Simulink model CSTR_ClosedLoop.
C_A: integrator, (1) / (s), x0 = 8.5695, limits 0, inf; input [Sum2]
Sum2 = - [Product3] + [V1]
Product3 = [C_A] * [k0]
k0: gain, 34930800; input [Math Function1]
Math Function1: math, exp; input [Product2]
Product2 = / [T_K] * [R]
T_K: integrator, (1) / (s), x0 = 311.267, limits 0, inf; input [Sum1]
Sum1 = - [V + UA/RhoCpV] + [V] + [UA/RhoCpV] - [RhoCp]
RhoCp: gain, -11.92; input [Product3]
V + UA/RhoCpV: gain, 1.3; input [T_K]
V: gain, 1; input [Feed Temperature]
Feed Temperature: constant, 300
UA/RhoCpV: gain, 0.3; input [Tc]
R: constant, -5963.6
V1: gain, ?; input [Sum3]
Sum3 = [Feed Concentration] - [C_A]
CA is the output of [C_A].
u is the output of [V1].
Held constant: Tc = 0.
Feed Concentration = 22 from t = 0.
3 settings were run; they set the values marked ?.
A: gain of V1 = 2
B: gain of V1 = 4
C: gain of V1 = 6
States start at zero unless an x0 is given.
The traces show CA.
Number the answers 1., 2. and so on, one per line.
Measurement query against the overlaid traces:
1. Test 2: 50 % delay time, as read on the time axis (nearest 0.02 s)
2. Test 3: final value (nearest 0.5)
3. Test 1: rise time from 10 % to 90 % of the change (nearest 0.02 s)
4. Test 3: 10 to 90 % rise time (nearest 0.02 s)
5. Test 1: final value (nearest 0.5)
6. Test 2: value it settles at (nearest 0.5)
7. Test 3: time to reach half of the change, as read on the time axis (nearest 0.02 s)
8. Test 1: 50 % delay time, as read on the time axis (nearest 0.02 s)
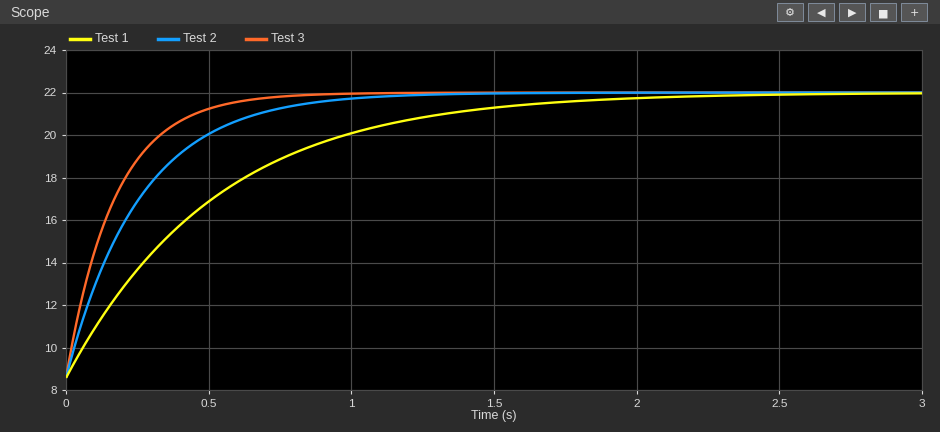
1. 0.18 s
2. 22.0
3. 1.12 s
4. 0.38 s
5. 22.0
6. 22.0
7. 0.12 s
8. 0.36 s
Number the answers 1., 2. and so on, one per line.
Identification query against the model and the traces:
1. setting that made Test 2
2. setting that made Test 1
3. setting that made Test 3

1. B
2. A
3. C
